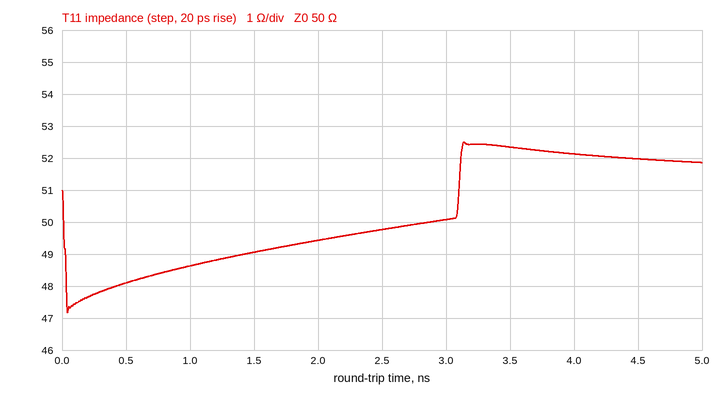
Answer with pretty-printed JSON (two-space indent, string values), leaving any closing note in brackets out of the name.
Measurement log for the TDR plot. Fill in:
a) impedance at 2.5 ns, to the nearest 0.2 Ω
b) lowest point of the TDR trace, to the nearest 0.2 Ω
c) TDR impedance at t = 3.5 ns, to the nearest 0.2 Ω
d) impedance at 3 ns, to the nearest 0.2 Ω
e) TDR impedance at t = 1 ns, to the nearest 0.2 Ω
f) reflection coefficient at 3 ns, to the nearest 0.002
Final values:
{
  "impedance at 2.5 ns, to the nearest 0.2 Ω": "49.8 Ω",
  "lowest point of the TDR trace, to the nearest 0.2 Ω": "47.2 Ω",
  "TDR impedance at t = 3.5 ns, to the nearest 0.2 Ω": "52.4 Ω",
  "impedance at 3 ns, to the nearest 0.2 Ω": "50.0 Ω",
  "TDR impedance at t = 1 ns, to the nearest 0.2 Ω": "48.6 Ω",
  "reflection coefficient at 3 ns, to the nearest 0.002": "0.000"
}
